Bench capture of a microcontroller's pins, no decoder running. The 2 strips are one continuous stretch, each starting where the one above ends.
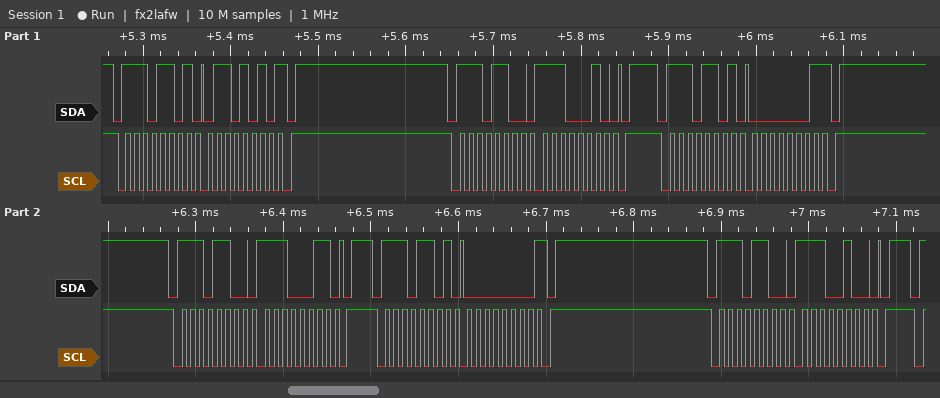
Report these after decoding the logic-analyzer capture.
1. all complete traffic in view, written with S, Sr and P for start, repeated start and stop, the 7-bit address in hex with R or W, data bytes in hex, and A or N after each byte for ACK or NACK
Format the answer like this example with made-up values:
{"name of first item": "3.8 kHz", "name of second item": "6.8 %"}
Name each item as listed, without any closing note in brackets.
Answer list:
{"all complete traffic in view, written with S, Sr and P for start, repeated start and stop, the 7-bit address in hex with R or W, data bytes in hex, and A or N after each byte for ACK or NACK": "S 76R A 6A N P S 76W A E2 A P S 76R A 01 N P S 76W A E3 A P S 76R A 00 N P S 76W A E4 A P"}
